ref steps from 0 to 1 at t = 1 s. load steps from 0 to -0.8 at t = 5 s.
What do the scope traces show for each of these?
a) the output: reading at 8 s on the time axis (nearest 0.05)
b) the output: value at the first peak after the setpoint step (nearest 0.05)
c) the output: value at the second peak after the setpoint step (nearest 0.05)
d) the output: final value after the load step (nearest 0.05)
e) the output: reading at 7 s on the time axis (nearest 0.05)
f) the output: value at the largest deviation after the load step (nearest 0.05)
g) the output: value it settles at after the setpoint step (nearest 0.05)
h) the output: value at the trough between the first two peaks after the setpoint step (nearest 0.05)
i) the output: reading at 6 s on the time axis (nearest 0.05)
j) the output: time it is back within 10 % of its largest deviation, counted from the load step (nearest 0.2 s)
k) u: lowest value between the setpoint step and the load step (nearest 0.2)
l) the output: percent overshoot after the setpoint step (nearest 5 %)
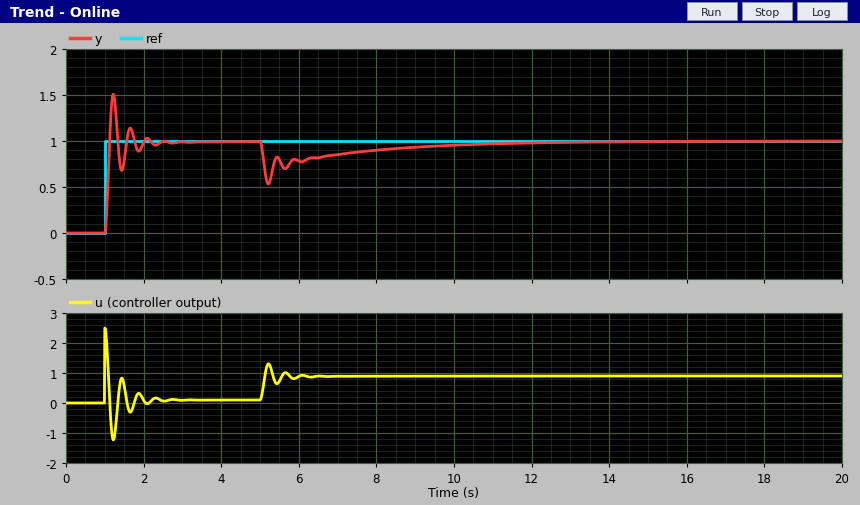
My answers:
0.90
1.50
1.15
1.00
0.85
0.55
1.00
0.70
0.80
5.0 s
-1.2
50 %
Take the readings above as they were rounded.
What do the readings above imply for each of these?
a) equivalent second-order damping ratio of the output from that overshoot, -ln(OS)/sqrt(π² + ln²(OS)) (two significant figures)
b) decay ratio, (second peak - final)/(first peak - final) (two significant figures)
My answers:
0.22
0.30
